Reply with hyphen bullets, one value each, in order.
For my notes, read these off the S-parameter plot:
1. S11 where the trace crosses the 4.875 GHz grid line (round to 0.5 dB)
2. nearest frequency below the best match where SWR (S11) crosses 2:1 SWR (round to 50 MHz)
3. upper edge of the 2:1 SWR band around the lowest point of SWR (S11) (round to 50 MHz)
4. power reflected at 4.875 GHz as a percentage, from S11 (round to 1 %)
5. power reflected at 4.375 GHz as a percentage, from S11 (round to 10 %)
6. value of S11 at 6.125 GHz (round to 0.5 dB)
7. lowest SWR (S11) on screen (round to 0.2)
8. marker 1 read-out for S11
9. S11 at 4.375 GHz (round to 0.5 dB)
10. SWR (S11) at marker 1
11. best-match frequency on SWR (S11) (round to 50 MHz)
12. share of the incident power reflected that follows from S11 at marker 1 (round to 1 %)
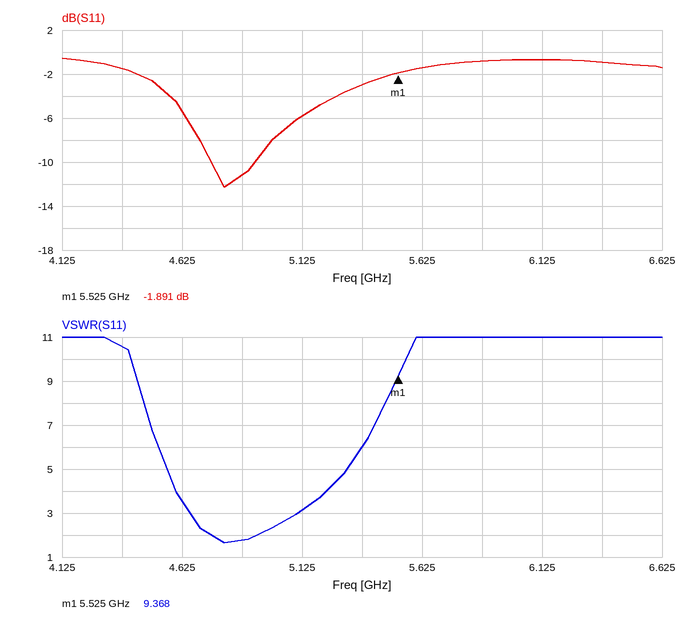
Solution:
- -11.0 dB
- 4.75 GHz
- 4.95 GHz
- 8 %
- 70 %
- -0.5 dB
- 1.6
- -1.891 dB
- -1.5 dB
- 9.368
- 4.80 GHz
- 65 %
